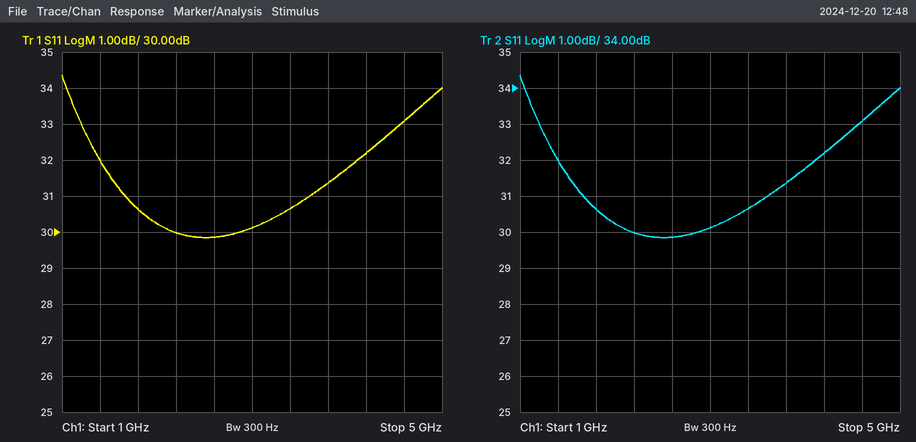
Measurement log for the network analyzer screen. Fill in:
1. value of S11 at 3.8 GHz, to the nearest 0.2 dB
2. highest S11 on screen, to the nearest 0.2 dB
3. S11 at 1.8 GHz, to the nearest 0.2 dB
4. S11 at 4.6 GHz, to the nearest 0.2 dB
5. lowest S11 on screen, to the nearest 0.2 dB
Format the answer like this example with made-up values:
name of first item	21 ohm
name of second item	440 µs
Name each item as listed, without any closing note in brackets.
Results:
value of S11 at 3.8 GHz, to the nearest 0.2 dB	31.4 dB
highest S11 on screen, to the nearest 0.2 dB	34.4 dB
S11 at 1.8 GHz, to the nearest 0.2 dB	30.6 dB
S11 at 4.6 GHz, to the nearest 0.2 dB	33.0 dB
lowest S11 on screen, to the nearest 0.2 dB	29.8 dB
